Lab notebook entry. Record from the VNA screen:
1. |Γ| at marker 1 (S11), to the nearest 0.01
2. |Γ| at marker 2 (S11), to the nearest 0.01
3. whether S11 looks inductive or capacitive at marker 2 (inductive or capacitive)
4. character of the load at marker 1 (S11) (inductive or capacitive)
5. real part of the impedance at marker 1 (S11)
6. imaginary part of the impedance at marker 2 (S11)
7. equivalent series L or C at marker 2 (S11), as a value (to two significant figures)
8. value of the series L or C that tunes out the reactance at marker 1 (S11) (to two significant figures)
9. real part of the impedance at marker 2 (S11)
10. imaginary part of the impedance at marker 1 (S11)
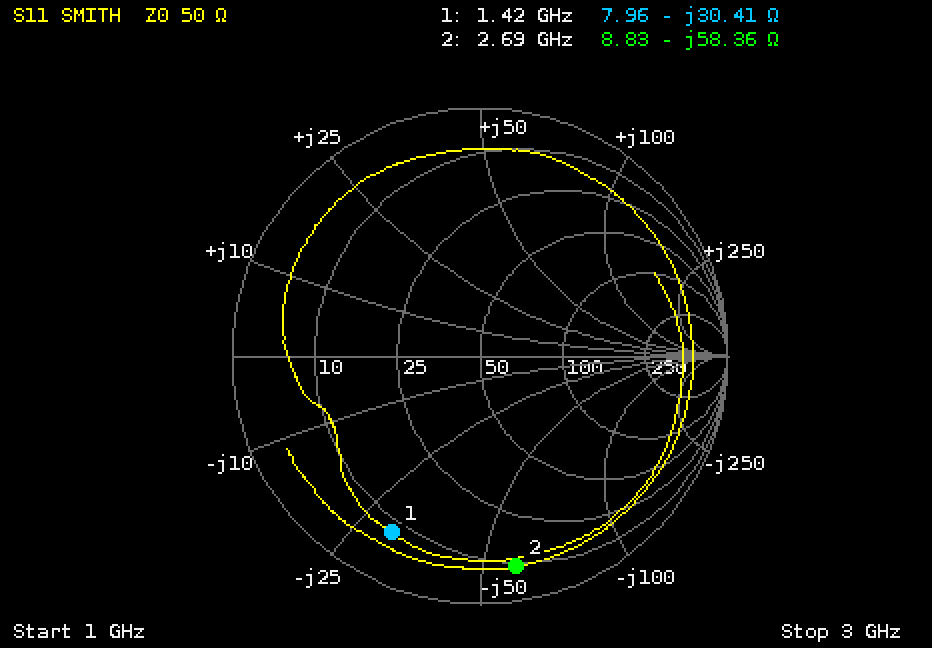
0.79
0.86
capacitive
capacitive
7.96 Ω
-58.36 Ω
1.0 pF
3.4 nH
8.83 Ω
-30.41 Ω
